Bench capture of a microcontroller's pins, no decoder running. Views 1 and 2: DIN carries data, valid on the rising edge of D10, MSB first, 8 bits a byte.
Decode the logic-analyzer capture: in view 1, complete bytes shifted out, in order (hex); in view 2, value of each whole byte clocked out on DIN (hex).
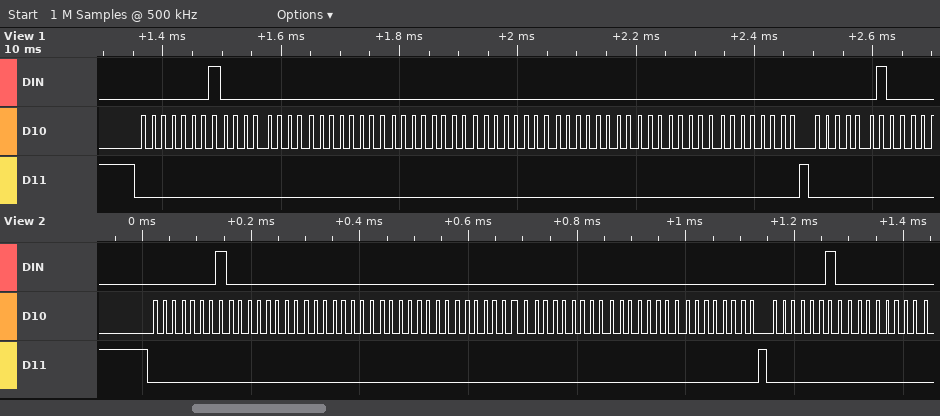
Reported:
01 00 00 00 00 00 00 00 02
0x01 0x00 0x00 0x00 0x00 0x00 0x00 0x00 0x02 0x00
